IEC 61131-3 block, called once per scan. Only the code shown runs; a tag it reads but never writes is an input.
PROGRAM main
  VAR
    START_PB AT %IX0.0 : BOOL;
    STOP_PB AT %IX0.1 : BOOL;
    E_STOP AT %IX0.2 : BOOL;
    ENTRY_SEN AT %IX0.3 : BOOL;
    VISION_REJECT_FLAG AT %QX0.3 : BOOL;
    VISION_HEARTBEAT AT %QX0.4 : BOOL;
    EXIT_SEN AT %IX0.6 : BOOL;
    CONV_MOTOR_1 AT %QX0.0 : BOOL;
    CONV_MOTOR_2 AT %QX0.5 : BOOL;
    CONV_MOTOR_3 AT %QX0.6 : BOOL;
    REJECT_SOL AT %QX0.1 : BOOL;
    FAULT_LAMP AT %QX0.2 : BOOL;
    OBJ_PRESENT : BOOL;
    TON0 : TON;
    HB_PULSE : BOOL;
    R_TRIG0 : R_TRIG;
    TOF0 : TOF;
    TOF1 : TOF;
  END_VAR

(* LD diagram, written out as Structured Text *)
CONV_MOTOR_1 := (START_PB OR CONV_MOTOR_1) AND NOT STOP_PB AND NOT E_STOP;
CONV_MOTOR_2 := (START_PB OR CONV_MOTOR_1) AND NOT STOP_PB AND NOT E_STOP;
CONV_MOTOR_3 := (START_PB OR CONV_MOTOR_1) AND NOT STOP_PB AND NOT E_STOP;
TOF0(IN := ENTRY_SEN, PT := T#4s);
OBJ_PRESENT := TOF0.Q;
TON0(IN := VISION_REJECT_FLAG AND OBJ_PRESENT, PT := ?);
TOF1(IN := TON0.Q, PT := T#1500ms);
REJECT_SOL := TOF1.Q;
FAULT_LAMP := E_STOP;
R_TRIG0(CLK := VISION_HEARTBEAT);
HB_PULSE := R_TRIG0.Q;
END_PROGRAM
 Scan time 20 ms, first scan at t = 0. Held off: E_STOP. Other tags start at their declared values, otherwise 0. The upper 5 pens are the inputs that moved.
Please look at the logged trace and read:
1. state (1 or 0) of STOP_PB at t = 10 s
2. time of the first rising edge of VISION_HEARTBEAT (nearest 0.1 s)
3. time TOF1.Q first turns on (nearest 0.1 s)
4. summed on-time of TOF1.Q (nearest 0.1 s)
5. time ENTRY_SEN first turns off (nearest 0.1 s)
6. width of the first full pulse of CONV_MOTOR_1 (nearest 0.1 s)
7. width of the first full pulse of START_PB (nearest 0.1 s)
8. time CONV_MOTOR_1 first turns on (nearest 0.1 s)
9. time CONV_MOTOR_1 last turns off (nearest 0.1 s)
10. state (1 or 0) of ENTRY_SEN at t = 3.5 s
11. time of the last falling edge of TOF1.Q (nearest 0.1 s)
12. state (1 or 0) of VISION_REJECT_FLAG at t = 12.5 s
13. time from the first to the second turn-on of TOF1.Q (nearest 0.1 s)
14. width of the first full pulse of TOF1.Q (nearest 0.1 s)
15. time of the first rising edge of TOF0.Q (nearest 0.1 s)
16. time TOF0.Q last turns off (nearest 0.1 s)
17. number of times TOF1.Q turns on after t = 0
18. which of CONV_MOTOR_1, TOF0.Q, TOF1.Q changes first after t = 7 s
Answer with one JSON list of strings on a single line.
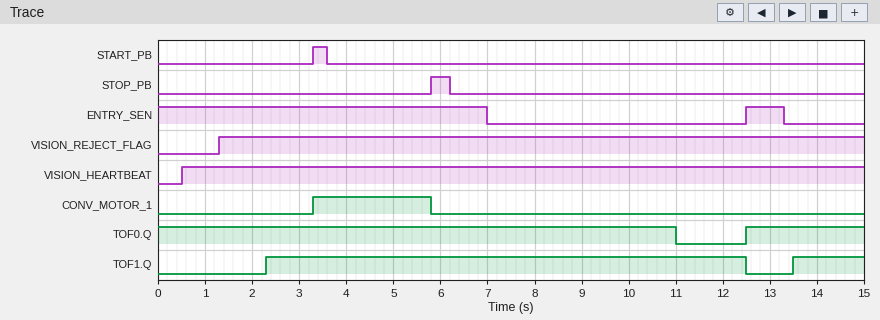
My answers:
["0", "0.5 s", "2.3 s", "11.7 s", "7.0 s", "2.5 s", "0.3 s", "3.3 s", "5.8 s", "1", "12.5 s", "1", "11.2 s", "10.2 s", "12.5 s", "11.0 s", "2", "TOF0.Q"]
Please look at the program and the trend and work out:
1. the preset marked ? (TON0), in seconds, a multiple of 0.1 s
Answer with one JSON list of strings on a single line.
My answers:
["1.0 s"]
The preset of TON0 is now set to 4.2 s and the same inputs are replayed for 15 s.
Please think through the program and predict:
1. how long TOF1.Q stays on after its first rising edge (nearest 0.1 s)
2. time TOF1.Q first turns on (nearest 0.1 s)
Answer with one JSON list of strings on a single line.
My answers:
["7.0 s", "5.5 s"]
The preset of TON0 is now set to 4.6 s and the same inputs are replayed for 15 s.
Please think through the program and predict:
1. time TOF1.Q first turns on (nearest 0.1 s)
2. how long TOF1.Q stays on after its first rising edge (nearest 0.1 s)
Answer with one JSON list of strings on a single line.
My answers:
["5.9 s", "6.6 s"]
